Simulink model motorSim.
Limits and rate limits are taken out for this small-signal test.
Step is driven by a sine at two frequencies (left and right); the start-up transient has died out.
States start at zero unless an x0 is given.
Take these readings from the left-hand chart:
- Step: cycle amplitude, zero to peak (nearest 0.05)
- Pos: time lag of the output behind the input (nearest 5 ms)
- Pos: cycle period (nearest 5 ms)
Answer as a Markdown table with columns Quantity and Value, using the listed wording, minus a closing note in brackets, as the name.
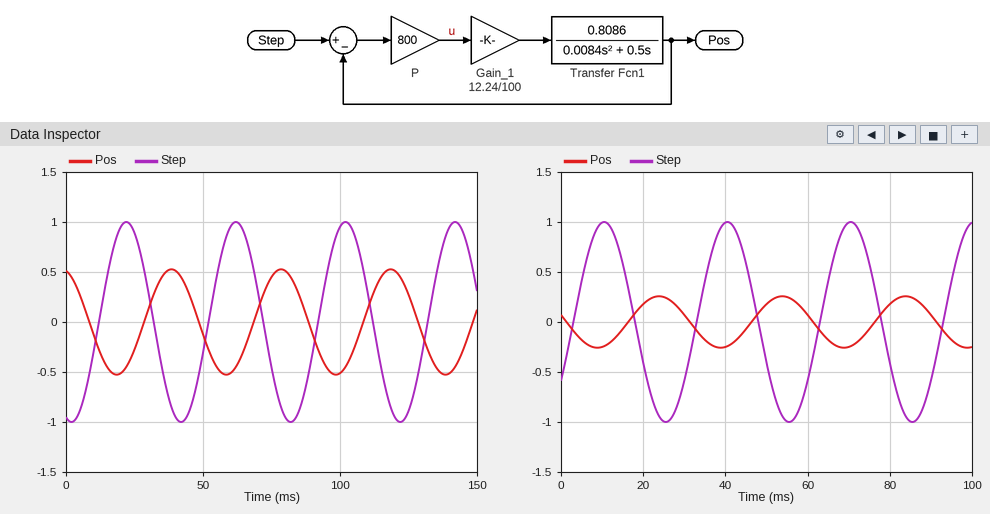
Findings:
| Quantity | Value |
|---|---|
| Step: cycle amplitude, zero to peak | 1.00 |
| Pos: time lag of the output behind the input | 15 ms |
| Pos: cycle period | 40 ms |
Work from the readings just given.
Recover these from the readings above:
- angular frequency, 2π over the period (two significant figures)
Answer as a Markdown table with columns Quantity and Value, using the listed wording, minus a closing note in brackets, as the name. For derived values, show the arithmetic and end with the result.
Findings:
| Quantity | Value |
|---|---|
| angular frequency, 2π over the period | 2π / 40 = 0.16 rad/ms |
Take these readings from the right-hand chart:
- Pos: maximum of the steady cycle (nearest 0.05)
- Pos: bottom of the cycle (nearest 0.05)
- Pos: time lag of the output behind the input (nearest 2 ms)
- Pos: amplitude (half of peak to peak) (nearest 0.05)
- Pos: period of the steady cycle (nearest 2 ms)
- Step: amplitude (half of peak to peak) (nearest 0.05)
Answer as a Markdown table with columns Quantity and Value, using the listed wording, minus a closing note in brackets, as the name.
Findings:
| Quantity | Value |
|---|---|
| Pos: maximum of the steady cycle | 0.25 |
| Pos: bottom of the cycle | -0.25 |
| Pos: time lag of the output behind the input | 14 ms |
| Pos: amplitude (half of peak to peak) | 0.25 |
| Pos: period of the steady cycle | 30 ms |
| Step: amplitude (half of peak to peak) | 1.00 |
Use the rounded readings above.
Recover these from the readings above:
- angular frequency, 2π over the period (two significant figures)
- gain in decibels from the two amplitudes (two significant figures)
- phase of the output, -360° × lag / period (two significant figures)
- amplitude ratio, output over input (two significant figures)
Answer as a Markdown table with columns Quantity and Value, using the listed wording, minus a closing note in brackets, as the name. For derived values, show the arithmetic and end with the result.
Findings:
| Quantity | Value |
|---|---|
| angular frequency, 2π over the period | 2π / 30 = 0.21 rad/ms |
| gain in decibels from the two amplitudes | 20 log10(0.25 / 1) = -12 dB |
| phase of the output, -360° × lag / period | -360 × 14 / 30 = -170° |
| amplitude ratio, output over input | 0.25 / 1 = 0.25 |
